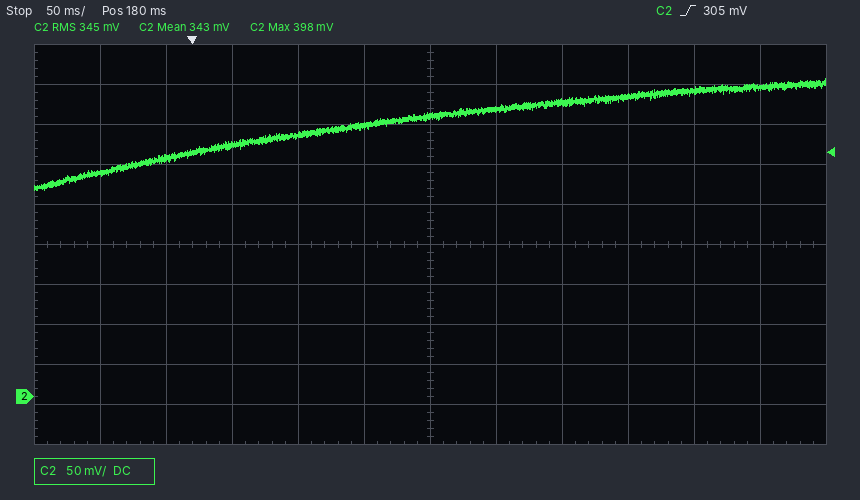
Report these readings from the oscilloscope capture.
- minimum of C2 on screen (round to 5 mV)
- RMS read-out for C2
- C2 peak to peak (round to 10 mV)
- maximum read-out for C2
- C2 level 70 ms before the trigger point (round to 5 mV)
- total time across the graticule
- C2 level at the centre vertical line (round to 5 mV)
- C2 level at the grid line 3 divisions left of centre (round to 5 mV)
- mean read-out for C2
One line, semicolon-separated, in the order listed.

260 mV; 345 mV; 140 mV; 398 mV; 280 mV; 600 ms; 350 mV; 315 mV; 343 mV
